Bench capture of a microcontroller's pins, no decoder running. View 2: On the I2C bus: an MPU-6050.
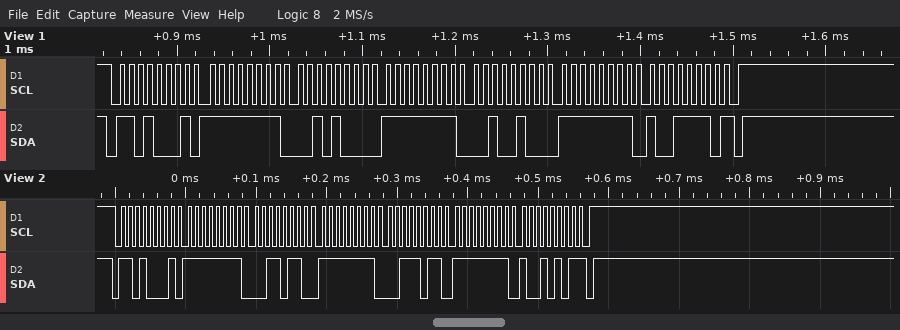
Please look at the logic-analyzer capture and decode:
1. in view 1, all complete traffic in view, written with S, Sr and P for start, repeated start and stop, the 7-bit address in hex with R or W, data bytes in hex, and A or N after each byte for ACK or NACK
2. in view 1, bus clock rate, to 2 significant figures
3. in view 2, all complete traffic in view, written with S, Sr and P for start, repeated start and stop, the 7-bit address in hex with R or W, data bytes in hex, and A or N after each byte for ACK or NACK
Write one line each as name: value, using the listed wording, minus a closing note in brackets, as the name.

in view 1, all complete traffic in view, written with S, Sr and P for start, repeated start and stop, the 7-bit address in hex with R or W, data bytes in hex, and A or N after each byte for ACK or NACK: S 68R A FF A 28 A FF A 24 A FF A 9E N P
in view 1, bus clock rate, to 2 significant figures: 100 kHz
in view 2, all complete traffic in view, written with S, Sr and P for start, repeated start and stop, the 7-bit address in hex with R or W, data bytes in hex, and A or N after each byte for ACK or NACK: S 68R A FF A 36 A FF A 3B A FF A 95 N P
